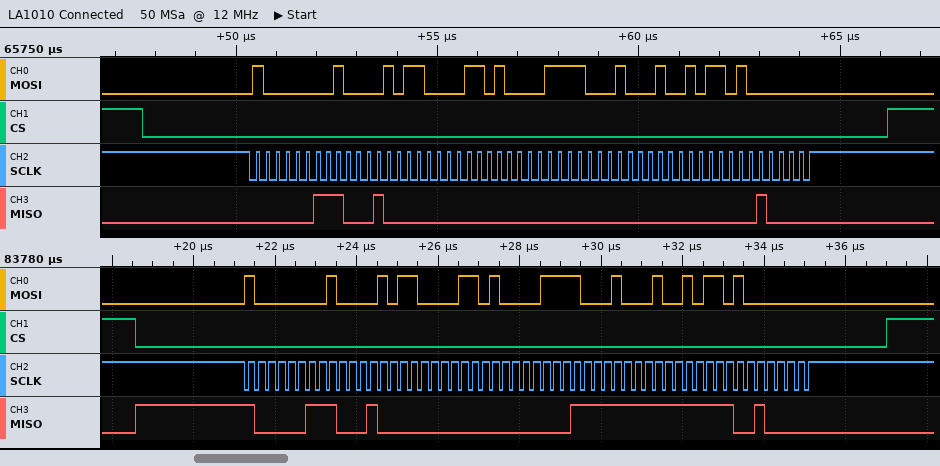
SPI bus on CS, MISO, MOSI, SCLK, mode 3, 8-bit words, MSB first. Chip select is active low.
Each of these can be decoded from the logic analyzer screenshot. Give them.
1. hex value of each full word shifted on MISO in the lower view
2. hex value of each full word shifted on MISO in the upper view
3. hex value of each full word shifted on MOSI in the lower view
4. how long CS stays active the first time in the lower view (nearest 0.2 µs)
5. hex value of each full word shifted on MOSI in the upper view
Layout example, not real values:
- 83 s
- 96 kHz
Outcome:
- 83, 88, 00, 00, FF, FF, 20
- 03, 88, 00, 00, 00, 00, 20
- 80, 85, 86, 87, 88, 96, 80
- 18.4 µs
- 80, 85, 86, 87, 88, 96, 80
